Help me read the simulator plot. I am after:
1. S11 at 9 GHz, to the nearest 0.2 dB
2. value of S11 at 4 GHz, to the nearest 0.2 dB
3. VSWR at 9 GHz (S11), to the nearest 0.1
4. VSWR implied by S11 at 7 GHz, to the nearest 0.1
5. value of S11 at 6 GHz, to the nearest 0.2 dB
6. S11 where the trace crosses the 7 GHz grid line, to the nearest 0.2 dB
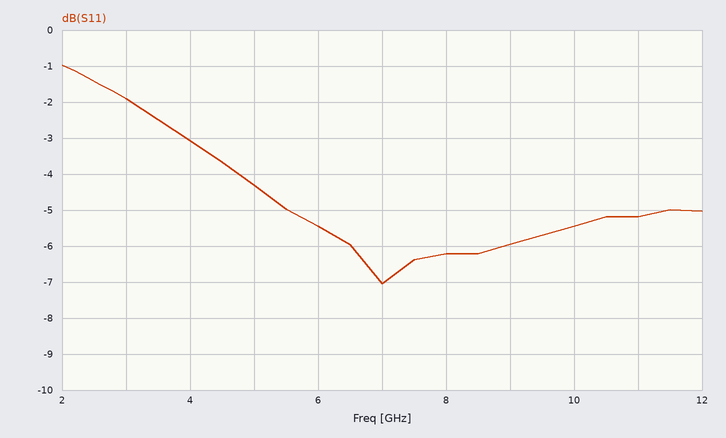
-6.0 dB
-3.0 dB
3.0
2.6
-5.4 dB
-7.0 dB
